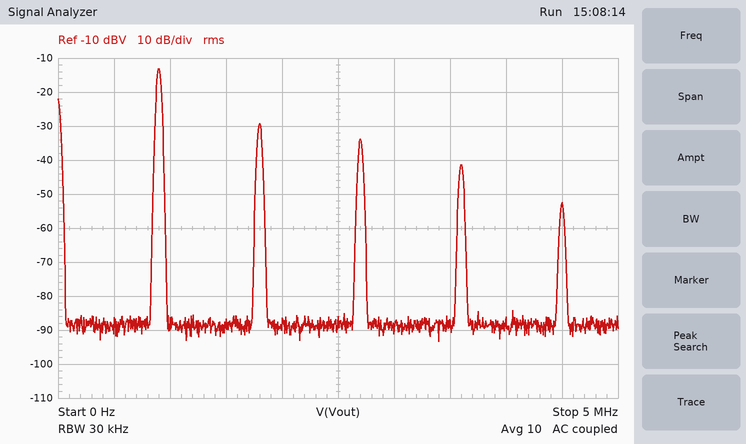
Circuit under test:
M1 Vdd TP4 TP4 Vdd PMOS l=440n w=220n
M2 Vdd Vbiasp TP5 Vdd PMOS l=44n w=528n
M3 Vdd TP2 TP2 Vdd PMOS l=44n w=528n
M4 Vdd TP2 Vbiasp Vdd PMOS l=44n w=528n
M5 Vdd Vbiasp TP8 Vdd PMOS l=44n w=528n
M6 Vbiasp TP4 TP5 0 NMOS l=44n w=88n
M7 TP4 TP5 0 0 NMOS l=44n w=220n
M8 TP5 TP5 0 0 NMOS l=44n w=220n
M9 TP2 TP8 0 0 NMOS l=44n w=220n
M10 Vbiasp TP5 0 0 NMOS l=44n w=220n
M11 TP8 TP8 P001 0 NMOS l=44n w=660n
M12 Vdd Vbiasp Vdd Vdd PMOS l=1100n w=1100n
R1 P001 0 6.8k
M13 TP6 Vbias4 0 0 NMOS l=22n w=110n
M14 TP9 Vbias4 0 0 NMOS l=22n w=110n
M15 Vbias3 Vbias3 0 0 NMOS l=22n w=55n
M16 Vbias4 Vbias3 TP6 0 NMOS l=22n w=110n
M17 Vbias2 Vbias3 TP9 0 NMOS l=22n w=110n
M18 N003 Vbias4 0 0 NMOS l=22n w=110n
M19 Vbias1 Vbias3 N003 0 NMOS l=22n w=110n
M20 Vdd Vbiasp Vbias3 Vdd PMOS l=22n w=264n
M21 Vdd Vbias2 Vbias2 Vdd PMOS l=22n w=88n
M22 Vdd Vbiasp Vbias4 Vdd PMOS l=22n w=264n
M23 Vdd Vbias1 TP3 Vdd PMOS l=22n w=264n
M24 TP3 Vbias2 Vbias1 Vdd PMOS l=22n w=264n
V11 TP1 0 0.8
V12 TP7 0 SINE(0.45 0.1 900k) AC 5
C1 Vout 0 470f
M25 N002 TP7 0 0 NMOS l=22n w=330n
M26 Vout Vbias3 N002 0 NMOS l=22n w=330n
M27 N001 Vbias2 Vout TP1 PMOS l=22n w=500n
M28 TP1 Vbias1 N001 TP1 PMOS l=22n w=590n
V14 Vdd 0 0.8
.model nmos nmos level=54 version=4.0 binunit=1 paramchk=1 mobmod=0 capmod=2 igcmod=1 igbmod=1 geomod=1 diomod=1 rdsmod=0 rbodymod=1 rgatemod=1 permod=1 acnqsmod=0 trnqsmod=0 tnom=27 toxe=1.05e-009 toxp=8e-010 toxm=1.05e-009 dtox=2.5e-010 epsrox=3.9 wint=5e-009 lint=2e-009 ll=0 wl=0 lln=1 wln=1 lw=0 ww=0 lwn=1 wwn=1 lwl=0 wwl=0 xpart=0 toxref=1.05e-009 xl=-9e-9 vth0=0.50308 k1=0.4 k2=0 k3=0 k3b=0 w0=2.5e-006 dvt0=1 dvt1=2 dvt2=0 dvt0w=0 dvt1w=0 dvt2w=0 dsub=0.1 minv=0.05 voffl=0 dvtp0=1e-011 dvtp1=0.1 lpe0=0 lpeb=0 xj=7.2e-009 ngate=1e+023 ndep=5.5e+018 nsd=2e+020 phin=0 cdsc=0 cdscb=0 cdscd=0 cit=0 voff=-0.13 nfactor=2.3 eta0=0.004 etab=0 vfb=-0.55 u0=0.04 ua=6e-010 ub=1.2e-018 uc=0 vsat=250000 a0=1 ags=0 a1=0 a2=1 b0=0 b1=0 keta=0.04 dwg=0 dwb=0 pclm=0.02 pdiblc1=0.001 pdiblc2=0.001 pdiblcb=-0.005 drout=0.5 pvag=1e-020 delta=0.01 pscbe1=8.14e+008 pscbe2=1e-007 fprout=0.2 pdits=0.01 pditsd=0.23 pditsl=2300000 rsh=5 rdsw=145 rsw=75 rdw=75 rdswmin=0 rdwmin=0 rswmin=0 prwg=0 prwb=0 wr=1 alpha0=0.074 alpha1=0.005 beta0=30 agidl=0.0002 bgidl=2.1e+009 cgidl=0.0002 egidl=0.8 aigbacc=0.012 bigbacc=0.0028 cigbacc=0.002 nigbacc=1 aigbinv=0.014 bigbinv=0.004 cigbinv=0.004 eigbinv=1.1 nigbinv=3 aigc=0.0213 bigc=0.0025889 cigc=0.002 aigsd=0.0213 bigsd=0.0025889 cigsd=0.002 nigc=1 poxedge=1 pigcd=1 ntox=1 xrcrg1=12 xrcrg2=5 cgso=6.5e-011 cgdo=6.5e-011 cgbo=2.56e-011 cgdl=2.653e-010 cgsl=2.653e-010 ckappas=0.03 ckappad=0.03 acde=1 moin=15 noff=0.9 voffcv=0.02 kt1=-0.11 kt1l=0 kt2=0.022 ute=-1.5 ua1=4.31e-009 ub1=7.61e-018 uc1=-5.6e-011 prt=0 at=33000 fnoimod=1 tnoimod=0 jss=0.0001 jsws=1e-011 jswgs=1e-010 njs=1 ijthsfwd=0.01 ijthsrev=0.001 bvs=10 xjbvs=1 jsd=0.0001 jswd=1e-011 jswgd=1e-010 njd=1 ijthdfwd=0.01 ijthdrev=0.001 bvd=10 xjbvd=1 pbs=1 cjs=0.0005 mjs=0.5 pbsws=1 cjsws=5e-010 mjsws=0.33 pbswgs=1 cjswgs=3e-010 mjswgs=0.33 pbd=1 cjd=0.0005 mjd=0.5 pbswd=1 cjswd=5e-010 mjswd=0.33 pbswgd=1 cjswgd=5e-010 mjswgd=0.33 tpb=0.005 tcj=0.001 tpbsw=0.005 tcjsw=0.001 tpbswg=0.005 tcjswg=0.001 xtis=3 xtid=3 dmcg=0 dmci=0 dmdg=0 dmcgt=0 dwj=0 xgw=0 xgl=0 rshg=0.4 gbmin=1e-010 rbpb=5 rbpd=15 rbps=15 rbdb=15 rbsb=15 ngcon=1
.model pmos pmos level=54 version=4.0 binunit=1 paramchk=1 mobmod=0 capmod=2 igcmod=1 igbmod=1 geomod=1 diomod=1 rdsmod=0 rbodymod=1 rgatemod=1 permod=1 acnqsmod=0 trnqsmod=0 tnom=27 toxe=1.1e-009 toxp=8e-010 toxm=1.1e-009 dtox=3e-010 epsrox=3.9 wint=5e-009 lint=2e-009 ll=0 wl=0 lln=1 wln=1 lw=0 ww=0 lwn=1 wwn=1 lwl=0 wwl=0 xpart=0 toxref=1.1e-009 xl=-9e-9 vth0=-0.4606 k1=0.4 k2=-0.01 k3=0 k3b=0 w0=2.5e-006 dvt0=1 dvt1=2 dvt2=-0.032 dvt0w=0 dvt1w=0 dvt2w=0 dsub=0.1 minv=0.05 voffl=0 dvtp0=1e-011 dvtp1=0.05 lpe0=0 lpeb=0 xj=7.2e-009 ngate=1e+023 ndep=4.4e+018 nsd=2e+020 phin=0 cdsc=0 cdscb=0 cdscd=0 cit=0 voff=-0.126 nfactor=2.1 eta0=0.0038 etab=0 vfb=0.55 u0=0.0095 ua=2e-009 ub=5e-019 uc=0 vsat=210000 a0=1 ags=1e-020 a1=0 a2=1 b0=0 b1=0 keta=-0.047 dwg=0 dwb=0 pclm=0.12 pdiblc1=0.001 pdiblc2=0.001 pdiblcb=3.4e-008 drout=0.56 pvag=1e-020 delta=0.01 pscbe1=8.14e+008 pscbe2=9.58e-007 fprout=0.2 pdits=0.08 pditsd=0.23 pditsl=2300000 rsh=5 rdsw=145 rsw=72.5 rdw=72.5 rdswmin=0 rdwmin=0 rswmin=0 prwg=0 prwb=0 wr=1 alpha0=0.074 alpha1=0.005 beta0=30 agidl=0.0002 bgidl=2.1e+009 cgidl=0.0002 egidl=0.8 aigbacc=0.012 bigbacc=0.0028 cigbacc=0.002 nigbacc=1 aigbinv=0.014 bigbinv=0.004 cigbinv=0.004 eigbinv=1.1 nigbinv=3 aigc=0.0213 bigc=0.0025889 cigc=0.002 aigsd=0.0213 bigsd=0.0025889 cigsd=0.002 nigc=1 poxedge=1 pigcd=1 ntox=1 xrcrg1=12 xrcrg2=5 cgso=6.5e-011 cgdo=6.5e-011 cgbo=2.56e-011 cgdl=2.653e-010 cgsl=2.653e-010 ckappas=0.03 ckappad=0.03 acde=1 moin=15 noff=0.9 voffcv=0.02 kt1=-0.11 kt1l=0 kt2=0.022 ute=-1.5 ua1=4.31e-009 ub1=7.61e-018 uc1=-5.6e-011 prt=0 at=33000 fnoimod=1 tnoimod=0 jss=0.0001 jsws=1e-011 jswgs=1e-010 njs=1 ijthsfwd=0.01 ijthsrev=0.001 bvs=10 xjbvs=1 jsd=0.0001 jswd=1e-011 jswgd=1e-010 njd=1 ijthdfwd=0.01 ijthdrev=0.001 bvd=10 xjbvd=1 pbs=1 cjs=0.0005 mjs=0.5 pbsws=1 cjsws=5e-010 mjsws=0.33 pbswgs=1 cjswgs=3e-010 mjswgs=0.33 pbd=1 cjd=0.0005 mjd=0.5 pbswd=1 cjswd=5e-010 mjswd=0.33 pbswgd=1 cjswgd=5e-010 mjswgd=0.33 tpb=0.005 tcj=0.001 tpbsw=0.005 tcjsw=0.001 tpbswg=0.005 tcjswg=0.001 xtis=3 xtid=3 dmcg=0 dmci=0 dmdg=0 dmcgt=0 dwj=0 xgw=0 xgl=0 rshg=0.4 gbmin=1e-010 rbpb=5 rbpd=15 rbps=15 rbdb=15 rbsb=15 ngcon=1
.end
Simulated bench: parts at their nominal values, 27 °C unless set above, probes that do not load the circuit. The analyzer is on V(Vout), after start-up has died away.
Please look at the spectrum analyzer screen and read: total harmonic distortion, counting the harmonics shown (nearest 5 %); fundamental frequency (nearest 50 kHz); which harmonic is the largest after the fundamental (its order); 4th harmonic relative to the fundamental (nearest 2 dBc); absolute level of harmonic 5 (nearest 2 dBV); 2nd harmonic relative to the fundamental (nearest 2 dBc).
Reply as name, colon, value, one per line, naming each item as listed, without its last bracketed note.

total harmonic distortion, counting the harmonics shown: 20 %
fundamental frequency: 900 kHz
which harmonic is the largest after the fundamental: 2
4th harmonic relative to the fundamental: -28 dBc
absolute level of harmonic 5: -52 dBV
2nd harmonic relative to the fundamental: -16 dBc
